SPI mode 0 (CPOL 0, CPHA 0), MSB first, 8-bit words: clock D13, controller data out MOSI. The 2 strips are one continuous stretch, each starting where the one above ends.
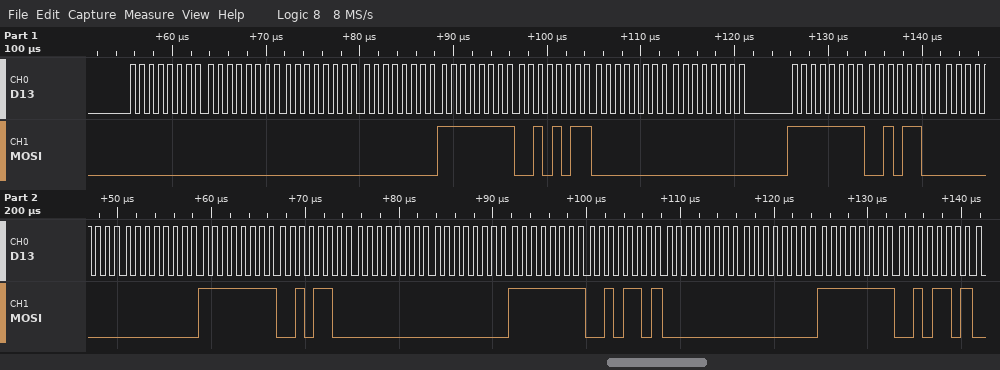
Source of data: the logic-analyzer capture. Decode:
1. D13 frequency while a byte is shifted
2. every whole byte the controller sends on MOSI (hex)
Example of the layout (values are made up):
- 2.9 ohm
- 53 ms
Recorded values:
- 1 MHz
- 00 00 00 00 FF 2B 00 00 FF 2C 00 00 FF 2C 00 00 FF 2D 00 00 FF 2D
